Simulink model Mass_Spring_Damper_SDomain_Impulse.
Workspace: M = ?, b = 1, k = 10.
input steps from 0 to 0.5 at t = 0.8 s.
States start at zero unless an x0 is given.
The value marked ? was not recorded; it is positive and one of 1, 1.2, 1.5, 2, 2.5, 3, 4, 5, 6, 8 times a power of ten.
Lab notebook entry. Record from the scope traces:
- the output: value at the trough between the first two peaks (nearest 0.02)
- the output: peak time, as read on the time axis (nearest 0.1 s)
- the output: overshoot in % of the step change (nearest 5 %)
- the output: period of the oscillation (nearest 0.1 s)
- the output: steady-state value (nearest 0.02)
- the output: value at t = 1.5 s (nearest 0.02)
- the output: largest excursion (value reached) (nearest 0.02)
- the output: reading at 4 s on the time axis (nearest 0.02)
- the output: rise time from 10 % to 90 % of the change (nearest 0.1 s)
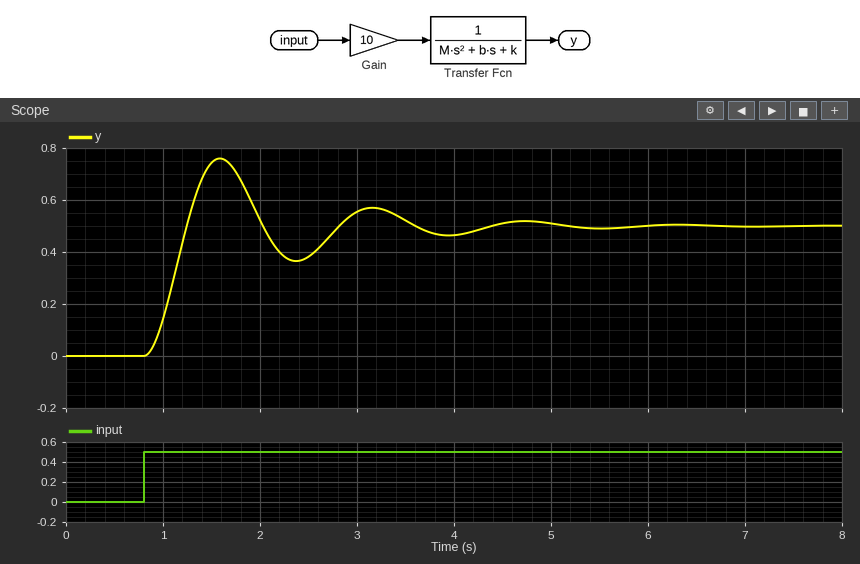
0.36
1.6 s
50 %
1.6 s
0.50
0.74
0.76
0.46
0.3 s
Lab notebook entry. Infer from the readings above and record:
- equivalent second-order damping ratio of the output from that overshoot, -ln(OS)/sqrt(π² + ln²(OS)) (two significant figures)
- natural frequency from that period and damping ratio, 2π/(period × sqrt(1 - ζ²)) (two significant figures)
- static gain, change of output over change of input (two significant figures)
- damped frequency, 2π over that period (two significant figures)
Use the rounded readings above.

0.22
4.0 rad/s
1.0
3.9 rad/s
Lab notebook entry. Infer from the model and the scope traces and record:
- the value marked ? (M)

0.6
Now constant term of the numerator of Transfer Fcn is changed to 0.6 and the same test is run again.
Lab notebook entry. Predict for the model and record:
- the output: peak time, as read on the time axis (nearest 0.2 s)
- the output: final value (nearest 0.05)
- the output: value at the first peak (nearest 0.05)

1.6 s
0.30
0.45
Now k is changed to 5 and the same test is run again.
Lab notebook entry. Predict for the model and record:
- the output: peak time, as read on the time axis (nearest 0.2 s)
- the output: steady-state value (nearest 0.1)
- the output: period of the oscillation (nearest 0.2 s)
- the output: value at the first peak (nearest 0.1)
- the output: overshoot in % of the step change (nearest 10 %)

2.0 s
1.0
2.2 s
1.4
40 %
